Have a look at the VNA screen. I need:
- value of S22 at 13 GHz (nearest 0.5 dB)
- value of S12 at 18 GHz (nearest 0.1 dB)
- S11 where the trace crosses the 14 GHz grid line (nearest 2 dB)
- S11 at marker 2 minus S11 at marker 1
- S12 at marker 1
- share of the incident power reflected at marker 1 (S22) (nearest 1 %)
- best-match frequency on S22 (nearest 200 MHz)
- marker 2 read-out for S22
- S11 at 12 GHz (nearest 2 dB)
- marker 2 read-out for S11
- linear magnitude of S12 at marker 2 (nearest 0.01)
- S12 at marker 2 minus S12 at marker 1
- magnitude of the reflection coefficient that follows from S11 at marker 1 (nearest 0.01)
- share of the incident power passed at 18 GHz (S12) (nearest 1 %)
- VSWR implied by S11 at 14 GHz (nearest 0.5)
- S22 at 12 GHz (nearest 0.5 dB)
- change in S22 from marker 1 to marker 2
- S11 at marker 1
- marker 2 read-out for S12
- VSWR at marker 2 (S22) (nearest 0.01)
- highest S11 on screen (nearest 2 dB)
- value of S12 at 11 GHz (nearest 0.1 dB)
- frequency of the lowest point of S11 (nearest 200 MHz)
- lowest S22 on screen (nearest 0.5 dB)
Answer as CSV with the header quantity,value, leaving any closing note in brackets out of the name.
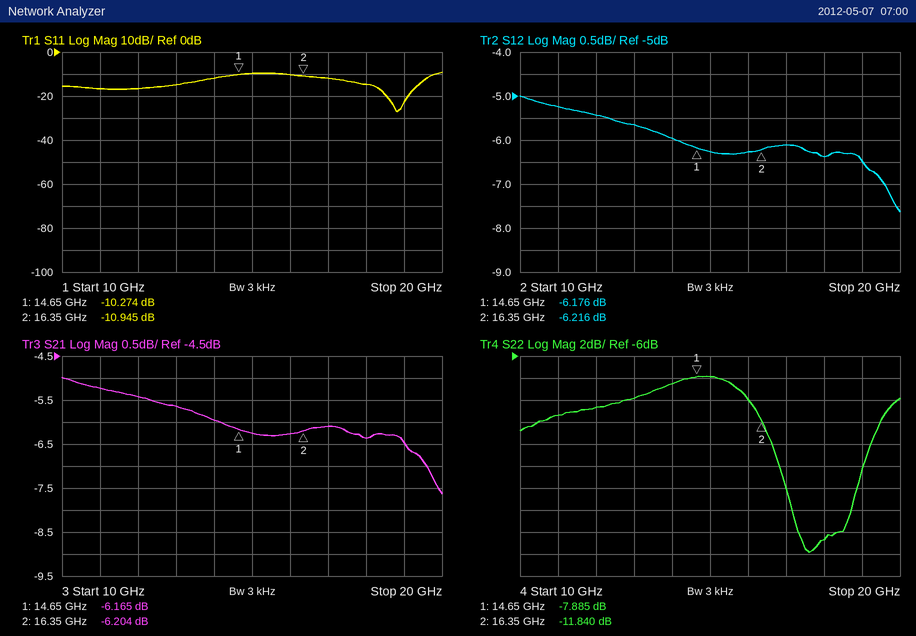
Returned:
quantity,value
value of S22 at 13 GHz,-10.0 dB
value of S12 at 18 GHz,-6.4 dB
S11 where the trace crosses the 14 GHz grid line,-12 dB
S11 at marker 2 minus S11 at marker 1,-0.671 dB
S12 at marker 1,-6.176 dB
share of the incident power reflected at marker 1 (S22),16 %
best-match frequency on S22,17.6 GHz
marker 2 read-out for S22,-11.840 dB
S11 at 12 GHz,-16 dB
marker 2 read-out for S11,-10.945 dB
linear magnitude of S12 at marker 2,0.49
S12 at marker 2 minus S12 at marker 1,-0.040 dB
magnitude of the reflection coefficient that follows from S11 at marker 1,0.31
share of the incident power passed at 18 GHz (S12),23 %
VSWR implied by S11 at 14 GHz,1.5
S22 at 12 GHz,-10.5 dB
change in S22 from marker 1 to marker 2,-3.955 dB
S11 at marker 1,-10.274 dB
marker 2 read-out for S12,-6.216 dB
VSWR at marker 2 (S22),1.69
highest S11 on screen,-10 dB
value of S12 at 11 GHz,-5.2 dB
frequency of the lowest point of S11,18.8 GHz
lowest S22 on screen,-24.0 dB
